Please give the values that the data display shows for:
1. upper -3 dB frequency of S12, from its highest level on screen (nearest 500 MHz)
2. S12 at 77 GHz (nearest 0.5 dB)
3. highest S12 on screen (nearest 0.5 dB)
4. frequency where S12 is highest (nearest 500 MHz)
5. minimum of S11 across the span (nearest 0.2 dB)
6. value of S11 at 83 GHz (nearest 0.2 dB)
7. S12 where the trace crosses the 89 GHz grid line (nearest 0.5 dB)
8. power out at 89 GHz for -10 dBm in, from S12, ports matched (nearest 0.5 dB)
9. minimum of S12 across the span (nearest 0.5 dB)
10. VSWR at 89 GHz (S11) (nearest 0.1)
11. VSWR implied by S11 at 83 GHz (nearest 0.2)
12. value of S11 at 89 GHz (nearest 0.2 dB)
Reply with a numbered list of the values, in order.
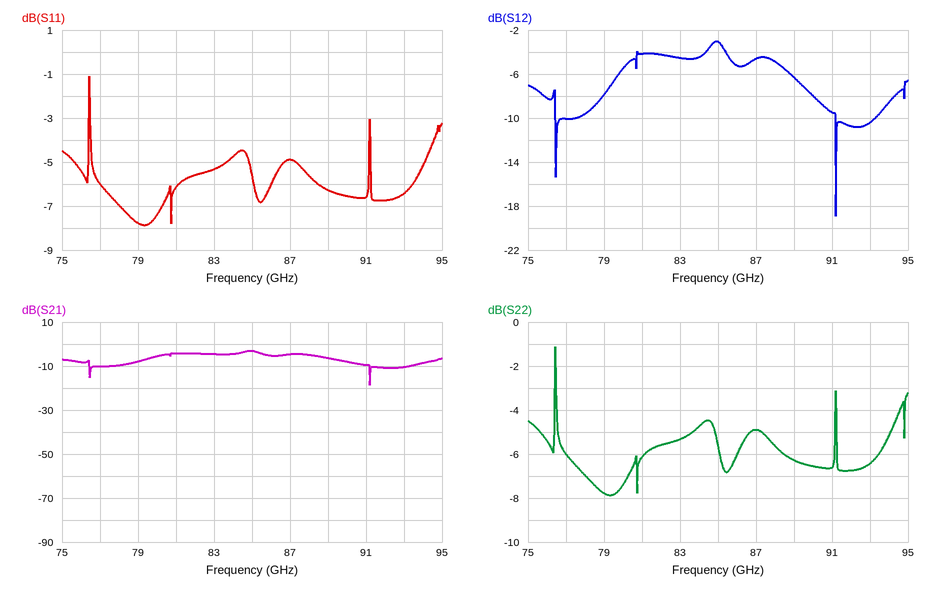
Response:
1. 89.0 GHz
2. -10.0 dB
3. -3.0 dB
4. 85.0 GHz
5. -7.8 dB
6. -5.4 dB
7. -6.5 dB
8. -16.5 dBm
9. -19.0 dB
10. 2.9
11. 3.4
12. -6.2 dB
